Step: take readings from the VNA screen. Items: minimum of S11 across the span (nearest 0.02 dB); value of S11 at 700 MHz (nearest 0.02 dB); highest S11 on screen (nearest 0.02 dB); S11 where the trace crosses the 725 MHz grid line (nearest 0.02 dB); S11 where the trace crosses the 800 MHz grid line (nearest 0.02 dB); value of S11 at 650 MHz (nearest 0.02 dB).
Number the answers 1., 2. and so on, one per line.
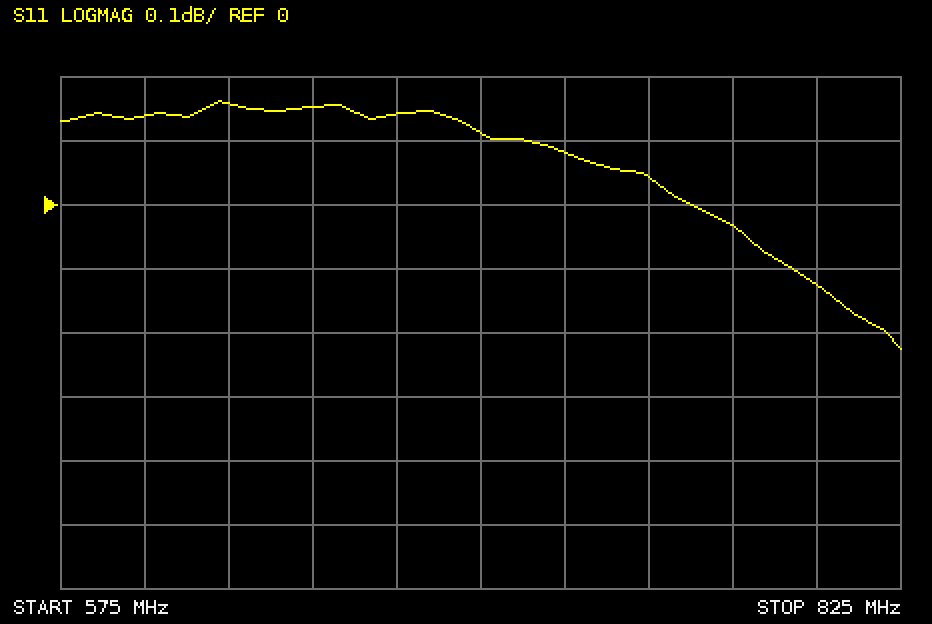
1. -0.22 dB
2. 0.12 dB
3. 0.16 dB
4. 0.08 dB
5. -0.12 dB
6. 0.16 dB
